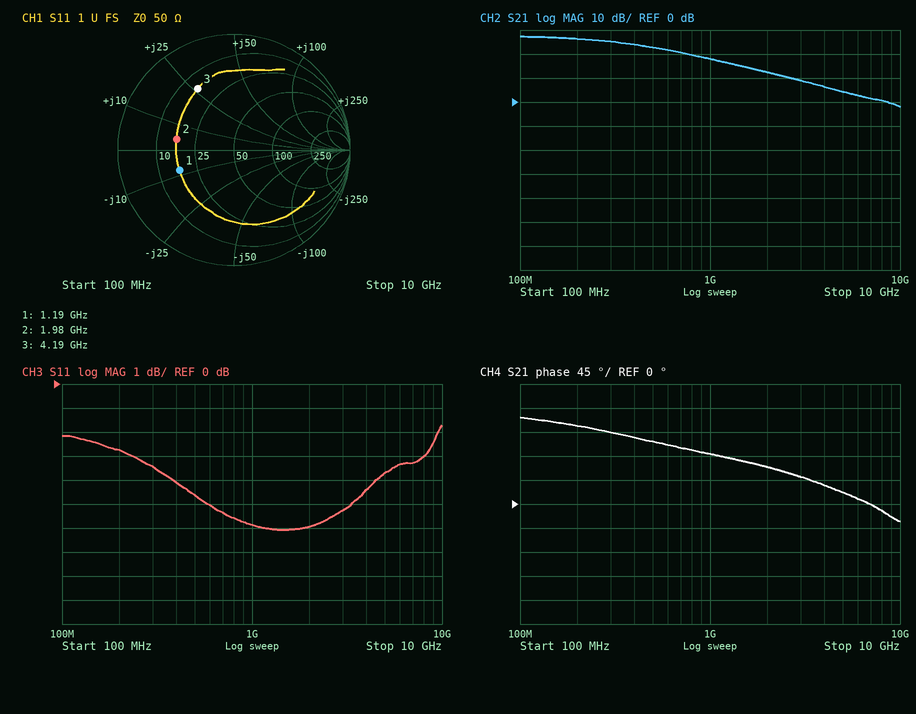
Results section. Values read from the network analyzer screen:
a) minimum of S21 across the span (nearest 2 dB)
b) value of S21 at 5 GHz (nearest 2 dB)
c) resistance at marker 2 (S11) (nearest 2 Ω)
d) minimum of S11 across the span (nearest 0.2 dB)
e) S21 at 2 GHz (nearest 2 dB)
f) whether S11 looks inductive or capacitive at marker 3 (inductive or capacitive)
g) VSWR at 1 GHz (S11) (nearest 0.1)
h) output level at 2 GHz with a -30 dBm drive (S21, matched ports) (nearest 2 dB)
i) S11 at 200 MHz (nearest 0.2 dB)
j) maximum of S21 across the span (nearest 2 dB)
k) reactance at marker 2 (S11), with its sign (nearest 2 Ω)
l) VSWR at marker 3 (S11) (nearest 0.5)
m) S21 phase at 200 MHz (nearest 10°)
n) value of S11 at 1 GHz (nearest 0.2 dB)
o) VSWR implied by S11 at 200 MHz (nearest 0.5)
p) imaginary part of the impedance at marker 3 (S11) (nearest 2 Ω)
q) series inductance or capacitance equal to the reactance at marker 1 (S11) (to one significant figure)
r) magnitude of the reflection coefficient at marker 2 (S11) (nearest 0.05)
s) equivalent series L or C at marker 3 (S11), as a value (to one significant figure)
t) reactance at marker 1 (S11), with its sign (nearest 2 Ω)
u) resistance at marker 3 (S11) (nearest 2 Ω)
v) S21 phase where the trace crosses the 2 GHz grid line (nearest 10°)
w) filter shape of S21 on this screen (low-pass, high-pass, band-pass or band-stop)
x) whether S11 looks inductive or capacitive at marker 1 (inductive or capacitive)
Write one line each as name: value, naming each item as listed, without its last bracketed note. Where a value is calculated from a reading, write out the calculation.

minimum of S21 across the span: -2 dB
value of S21 at 5 GHz: 4 dB
resistance at marker 2 (S11): 16 Ω
minimum of S11 across the span: -6.0 dB
S21 at 2 GHz: 12 dB
whether S11 looks inductive or capacitive at marker 3: inductive
VSWR at 1 GHz (S11): |Γ| = 10^(-5.8/20) = 0.5129; VSWR = (1 + 0.5129)/(1 − 0.5129) ≈ 3.1
output level at 2 GHz with a -30 dBm drive (S21, matched ports): -30 dBm + (12 dB) = -18 dBm
S11 at 200 MHz: -2.8 dB
maximum of S21 across the span: 28 dB
reactance at marker 2 (S11), with its sign: +4 Ω
VSWR at marker 3 (S11): 4.0
S21 phase at 200 MHz: 150°
value of S11 at 1 GHz: -5.8 dB
VSWR implied by S11 at 200 MHz: |Γ| = 10^(-2.8/20) = 0.7244; VSWR = (1 + 0.7244)/(1 − 0.7244) ≈ 6.26, so 6.5 to the nearest 0.5
imaginary part of the impedance at marker 3 (S11): +26 Ω
series inductance or capacitance equal to the reactance at marker 1 (S11): C = 1/(2π × 1.19 GHz × 8 Ω) ≈ 16.7 pF, so 20 pF to one significant figure
magnitude of the reflection coefficient at marker 2 (S11): 0.50
equivalent series L or C at marker 3 (S11), as a value: L = 26 Ω/(2π × 4.19 GHz) ≈ 1.0 nH
reactance at marker 1 (S11), with its sign: -8 Ω
resistance at marker 3 (S11): 16 Ω
S21 phase where the trace crosses the 2 GHz grid line: 70°
filter shape of S21 on this screen: low-pass
whether S11 looks inductive or capacitive at marker 1: capacitive
